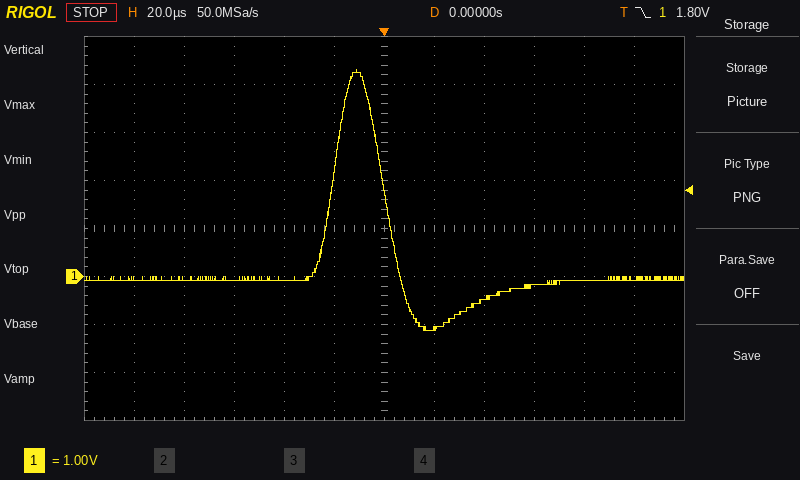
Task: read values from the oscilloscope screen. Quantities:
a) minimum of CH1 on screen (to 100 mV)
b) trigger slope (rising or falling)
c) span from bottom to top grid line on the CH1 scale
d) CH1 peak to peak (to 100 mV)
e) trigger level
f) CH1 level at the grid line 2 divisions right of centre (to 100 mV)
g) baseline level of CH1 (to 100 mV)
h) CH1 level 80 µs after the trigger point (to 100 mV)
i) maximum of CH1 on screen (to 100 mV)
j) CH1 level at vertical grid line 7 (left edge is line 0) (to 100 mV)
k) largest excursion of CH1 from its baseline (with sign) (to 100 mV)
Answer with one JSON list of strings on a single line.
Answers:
["-1.1 V", "falling", "8 V", "5.4 V", "1.80 V", "-400 mV", "-100 mV", "-100 mV", "4.3 V", "-1.1 V", "+4.4 V"]
